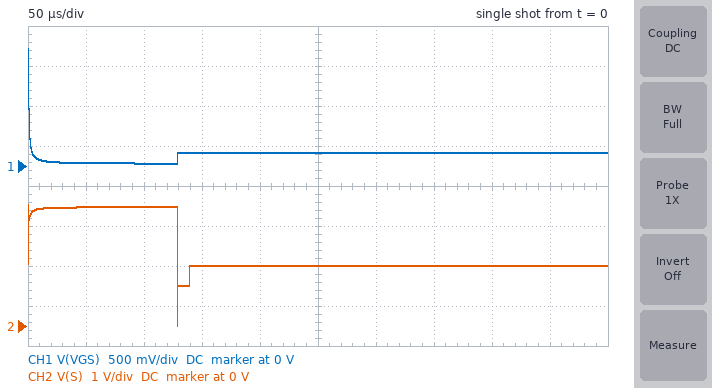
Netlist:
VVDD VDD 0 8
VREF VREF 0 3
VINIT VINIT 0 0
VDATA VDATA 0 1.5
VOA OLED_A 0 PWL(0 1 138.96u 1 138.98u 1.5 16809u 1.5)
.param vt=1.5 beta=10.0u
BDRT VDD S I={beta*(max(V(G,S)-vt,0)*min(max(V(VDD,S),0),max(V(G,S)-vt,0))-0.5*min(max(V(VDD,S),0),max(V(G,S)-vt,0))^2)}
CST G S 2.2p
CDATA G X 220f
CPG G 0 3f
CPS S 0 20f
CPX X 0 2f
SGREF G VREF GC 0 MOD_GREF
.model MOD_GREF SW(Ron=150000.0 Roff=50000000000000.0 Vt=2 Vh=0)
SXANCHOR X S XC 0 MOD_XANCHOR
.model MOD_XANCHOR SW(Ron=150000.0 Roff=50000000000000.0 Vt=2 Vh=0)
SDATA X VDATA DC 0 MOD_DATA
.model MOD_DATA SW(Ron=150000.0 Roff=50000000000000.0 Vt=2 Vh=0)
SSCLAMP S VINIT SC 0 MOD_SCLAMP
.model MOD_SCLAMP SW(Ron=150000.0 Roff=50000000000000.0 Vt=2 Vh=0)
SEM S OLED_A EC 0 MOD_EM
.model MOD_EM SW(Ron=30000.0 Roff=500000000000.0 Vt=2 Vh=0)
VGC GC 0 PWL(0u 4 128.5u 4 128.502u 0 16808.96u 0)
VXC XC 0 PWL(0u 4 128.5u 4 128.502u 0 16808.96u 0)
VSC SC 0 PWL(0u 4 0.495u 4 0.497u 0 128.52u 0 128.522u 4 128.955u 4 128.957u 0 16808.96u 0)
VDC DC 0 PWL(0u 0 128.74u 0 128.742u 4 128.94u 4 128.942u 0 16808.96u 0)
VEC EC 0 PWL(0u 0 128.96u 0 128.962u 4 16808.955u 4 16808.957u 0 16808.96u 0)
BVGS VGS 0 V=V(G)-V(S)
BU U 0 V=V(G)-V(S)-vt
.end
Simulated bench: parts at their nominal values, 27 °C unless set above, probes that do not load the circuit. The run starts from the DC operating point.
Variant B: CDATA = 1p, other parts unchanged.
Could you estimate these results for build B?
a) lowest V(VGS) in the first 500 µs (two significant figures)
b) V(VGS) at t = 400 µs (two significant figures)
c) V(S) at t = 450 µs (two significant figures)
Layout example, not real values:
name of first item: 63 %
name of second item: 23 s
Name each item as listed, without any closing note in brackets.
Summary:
lowest V(VGS) in the first 500 µs: 31 mV
V(VGS) at t = 400 µs: 320 mV
V(S) at t = 450 µs: 1.5 V
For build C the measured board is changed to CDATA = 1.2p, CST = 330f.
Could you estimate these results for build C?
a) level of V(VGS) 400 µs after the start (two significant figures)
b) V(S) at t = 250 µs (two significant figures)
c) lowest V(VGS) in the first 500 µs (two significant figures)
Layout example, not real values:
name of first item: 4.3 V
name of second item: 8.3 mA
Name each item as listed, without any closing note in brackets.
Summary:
level of V(VGS) 400 µs after the start: 810 mV
V(S) at t = 250 µs: 1.6 V
lowest V(VGS) in the first 500 µs: 28 mV
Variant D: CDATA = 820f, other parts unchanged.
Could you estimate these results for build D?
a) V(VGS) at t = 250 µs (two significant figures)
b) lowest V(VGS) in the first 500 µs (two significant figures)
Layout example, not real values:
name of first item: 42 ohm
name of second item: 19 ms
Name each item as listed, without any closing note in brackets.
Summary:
V(VGS) at t = 250 µs: 300 mV
lowest V(VGS) in the first 500 µs: 31 mV
